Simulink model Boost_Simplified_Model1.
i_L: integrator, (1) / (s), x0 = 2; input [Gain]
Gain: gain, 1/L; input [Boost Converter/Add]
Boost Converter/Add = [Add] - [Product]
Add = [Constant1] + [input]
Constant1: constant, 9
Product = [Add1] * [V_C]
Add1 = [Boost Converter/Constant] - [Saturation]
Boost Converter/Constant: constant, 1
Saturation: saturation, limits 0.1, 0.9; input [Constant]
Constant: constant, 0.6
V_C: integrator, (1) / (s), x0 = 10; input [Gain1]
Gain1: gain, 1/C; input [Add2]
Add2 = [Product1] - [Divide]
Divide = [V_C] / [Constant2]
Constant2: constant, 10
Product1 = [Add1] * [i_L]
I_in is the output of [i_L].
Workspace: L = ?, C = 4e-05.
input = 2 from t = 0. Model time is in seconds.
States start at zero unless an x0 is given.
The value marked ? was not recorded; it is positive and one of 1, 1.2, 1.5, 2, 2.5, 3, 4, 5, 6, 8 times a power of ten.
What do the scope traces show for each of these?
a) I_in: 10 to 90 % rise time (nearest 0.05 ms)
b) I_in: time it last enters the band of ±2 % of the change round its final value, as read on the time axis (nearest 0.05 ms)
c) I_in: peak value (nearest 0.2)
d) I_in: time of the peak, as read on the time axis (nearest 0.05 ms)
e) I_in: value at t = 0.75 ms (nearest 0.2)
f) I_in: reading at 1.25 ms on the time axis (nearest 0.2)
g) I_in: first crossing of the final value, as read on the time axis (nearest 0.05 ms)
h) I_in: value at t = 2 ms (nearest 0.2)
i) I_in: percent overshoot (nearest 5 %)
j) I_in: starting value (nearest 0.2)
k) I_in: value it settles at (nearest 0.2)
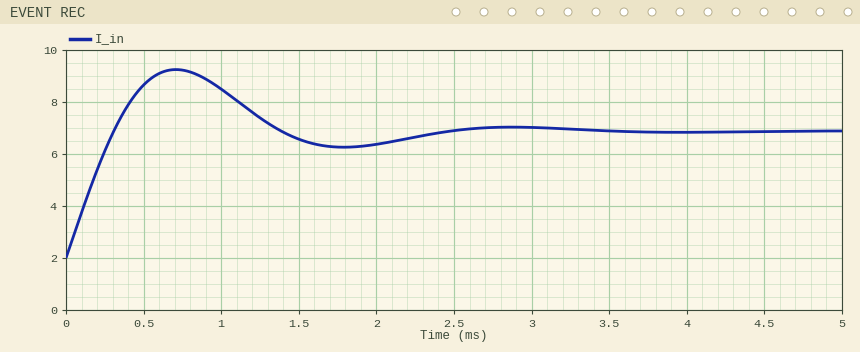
0.25 ms
3.20 ms
9.2
0.70 ms
9.2
7.4
0.30 ms
6.4
50 %
2.0
6.8
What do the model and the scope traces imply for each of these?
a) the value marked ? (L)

0.0004
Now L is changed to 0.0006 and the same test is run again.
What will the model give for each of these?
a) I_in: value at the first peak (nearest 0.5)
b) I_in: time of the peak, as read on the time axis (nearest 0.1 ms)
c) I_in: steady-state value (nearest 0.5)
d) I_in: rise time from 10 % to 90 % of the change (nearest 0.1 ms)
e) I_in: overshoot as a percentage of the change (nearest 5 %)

8.5
1.0 ms
7.0
0.4 ms
30 %
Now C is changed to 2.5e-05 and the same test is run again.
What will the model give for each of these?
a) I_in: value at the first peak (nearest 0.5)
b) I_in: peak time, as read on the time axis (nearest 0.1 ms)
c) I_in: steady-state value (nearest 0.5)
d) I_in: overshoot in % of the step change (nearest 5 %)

8.0
0.6 ms
7.0
25 %
